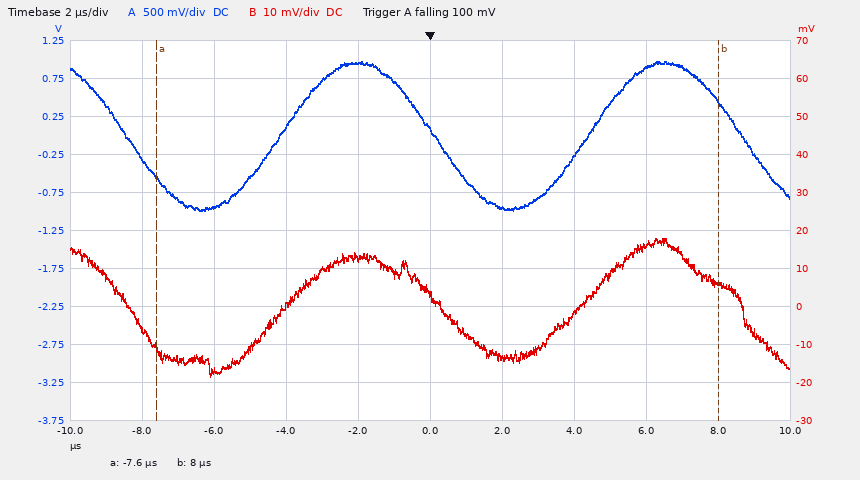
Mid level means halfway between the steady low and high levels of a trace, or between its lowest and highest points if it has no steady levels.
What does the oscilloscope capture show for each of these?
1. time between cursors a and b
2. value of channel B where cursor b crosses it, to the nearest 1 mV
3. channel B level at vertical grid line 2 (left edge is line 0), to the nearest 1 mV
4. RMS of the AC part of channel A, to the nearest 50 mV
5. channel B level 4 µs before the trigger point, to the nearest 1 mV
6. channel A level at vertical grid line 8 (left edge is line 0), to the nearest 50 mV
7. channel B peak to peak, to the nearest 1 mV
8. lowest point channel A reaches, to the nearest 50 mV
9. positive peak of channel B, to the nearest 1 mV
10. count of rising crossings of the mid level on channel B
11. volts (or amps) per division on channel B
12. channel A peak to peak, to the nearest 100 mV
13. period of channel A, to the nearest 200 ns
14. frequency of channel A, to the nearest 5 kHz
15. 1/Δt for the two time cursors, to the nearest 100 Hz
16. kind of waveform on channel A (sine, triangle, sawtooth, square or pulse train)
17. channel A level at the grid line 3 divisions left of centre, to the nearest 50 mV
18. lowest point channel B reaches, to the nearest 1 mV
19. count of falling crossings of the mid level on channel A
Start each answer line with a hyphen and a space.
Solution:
- 15.6 µs
- 6 mV
- -17 mV
- 700 mV
- 0 mV
- 900 mV
- 36 mV
- -1.00 V
- 18 mV
- 2
- 10 mV
- 2.00 V
- 8.6 µs
- 115 kHz
- 64.1 kHz
- sine
- -950 mV
- -18 mV
- 3
